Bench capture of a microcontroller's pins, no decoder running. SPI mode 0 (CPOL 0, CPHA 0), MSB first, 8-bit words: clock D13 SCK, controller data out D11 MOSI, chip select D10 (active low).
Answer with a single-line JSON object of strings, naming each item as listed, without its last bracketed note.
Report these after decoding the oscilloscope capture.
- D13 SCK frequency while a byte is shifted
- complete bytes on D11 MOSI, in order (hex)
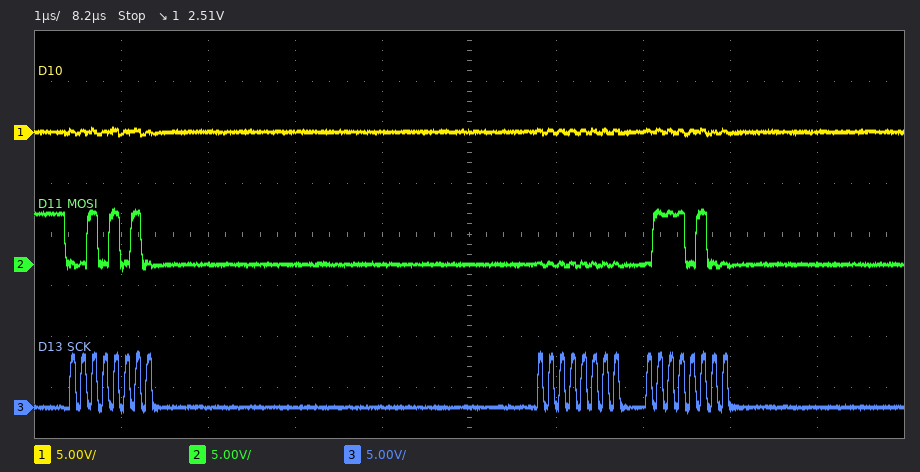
{"D13 SCK frequency while a byte is shifted": "8 MHz", "complete bytes on D11 MOSI, in order": "2A 00 74"}
